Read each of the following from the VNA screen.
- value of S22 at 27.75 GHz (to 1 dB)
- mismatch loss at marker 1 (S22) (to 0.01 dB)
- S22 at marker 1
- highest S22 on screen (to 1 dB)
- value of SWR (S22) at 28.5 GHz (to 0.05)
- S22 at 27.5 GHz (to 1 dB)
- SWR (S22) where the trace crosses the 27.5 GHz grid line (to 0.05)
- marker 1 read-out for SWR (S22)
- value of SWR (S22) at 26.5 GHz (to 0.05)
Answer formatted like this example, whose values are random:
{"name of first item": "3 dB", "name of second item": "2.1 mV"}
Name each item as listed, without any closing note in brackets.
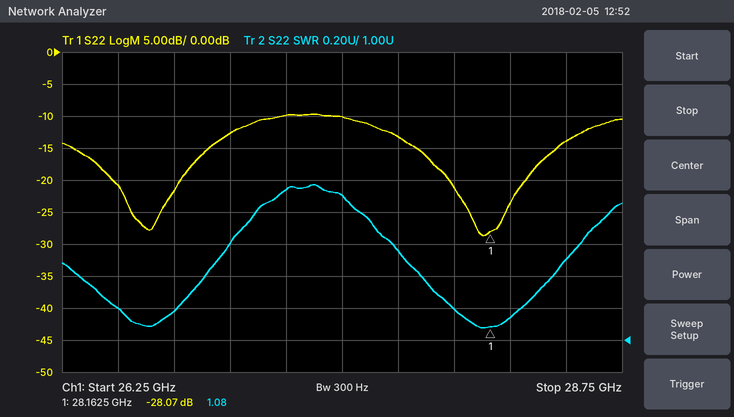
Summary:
{"value of S22 at 27.75 GHz": "-13 dB", "mismatch loss at marker 1 (S22)": "0.01 dB", "S22 at marker 1": "-28.07 dB", "highest S22 on screen": "-10 dB", "value of SWR (S22) at 28.5 GHz": "1.50", "S22 at 27.5 GHz": "-10 dB", "SWR (S22) where the trace crosses the 27.5 GHz grid line": "1.90", "marker 1 read-out for SWR": "1.08", "value of SWR (S22) at 26.5 GHz": "1.20"}
